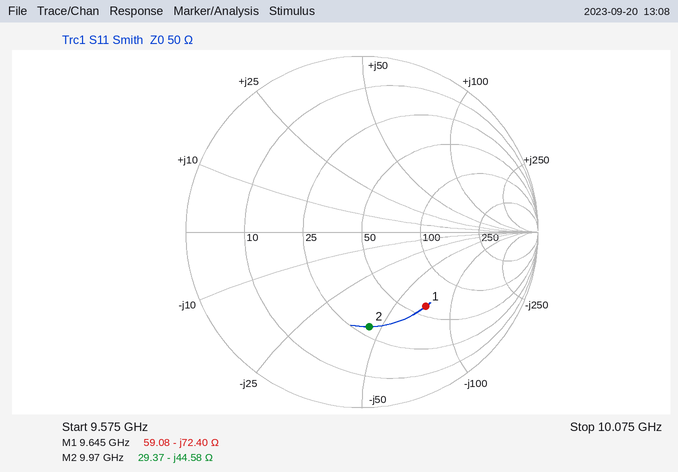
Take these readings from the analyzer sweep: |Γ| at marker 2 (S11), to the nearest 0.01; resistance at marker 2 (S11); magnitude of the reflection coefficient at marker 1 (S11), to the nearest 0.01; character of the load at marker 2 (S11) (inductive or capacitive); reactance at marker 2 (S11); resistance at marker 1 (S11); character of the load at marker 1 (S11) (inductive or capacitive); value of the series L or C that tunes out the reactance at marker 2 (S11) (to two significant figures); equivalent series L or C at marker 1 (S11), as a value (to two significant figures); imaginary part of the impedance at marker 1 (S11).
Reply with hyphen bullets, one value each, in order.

- 0.54
- 29.37 Ω
- 0.56
- capacitive
- -44.58 Ω
- 59.08 Ω
- capacitive
- 710 pH
- 230 fF
- -72.40 Ω
